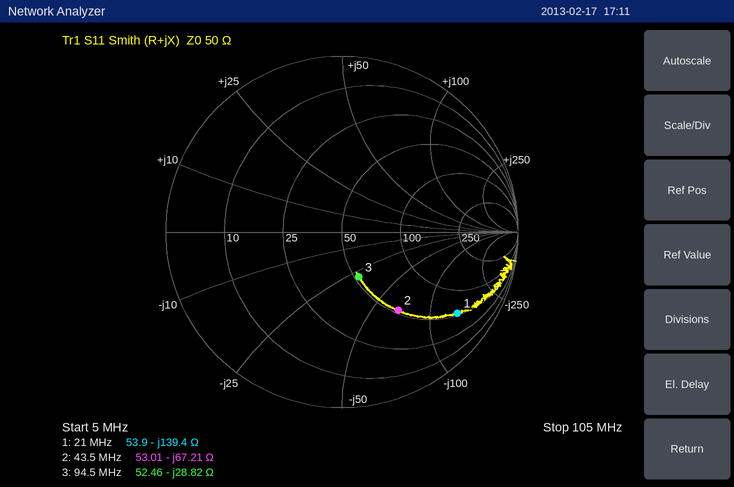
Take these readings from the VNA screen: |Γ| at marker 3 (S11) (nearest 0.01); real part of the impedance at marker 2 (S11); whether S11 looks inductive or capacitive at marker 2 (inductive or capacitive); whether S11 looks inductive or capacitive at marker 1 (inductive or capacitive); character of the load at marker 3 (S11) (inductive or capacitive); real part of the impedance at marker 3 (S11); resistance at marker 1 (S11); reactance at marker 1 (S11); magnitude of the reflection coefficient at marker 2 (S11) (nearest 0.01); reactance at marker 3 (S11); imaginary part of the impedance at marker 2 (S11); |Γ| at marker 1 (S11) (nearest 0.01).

0.27
53.01 Ω
capacitive
capacitive
capacitive
52.46 Ω
53.9 Ω
-139.4 Ω
0.55
-28.82 Ω
-67.21 Ω
0.80
